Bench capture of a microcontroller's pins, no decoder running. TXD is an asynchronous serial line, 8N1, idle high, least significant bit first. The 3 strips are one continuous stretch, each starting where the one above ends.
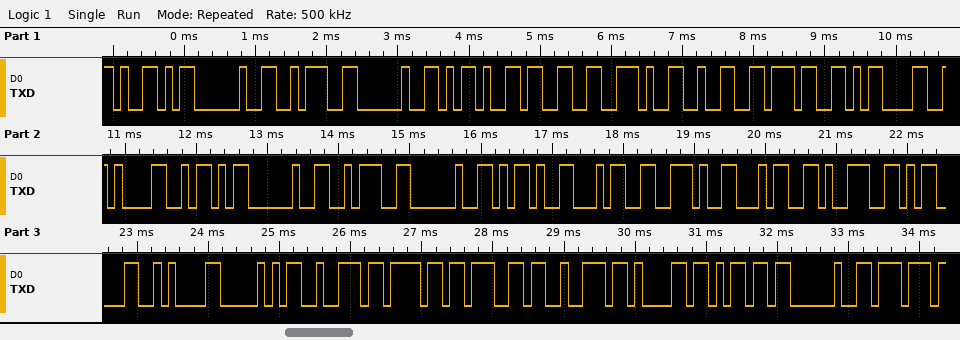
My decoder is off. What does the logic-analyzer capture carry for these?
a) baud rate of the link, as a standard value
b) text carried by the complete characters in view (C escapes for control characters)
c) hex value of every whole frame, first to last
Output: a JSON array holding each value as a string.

["9600 baud", "\"Y : -3.27\\r\\nZ : -4.49\\r\\nProgram w\"", "0x59 0x20 0x3A 0x20 0x2D 0x33 0x2E 0x32 0x37 0x0D 0x0A 0x5A 0x20 0x3A 0x20 0x2D 0x34 0x2E 0x34 0x39 0x0D 0x0A 0x50 0x72 0x6F 0x67 0x72 0x61 0x6D 0x20 0x77"]
